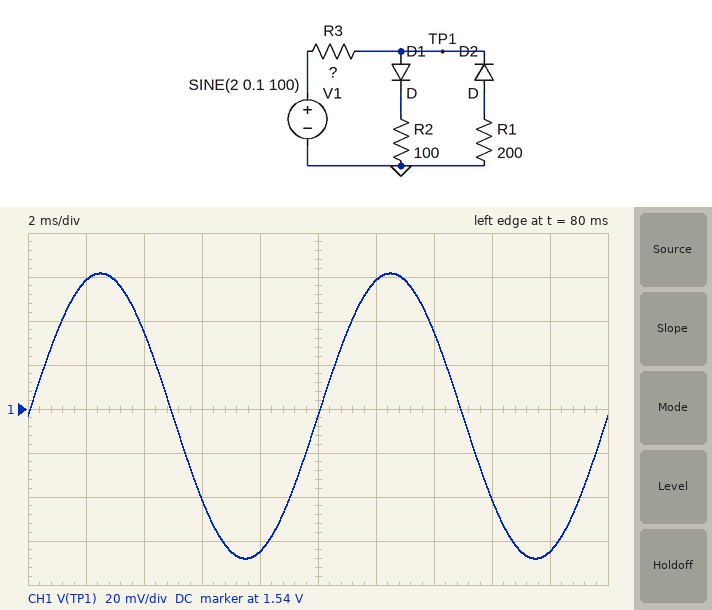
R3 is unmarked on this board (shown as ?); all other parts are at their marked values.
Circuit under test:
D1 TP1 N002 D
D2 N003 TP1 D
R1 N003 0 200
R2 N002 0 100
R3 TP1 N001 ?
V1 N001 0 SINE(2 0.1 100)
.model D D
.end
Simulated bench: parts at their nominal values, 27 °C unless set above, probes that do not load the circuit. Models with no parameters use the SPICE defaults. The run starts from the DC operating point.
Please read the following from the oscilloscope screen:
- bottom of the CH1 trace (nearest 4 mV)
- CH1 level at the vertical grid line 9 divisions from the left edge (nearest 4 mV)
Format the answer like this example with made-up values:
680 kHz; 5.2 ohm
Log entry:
1.472 V; 1.476 V
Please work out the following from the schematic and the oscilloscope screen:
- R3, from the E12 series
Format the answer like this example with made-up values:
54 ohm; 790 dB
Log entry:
56 Ω
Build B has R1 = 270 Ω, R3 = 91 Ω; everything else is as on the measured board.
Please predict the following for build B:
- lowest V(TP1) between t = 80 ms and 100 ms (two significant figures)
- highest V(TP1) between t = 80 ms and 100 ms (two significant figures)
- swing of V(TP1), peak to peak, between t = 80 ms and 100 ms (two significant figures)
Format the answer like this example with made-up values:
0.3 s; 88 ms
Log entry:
1.3 V; 1.4 V; 110 mV
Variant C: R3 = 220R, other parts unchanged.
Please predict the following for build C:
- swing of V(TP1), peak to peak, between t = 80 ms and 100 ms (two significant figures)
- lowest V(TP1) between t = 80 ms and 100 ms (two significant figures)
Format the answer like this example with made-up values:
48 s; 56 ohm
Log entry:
65 mV; 1.1 V
